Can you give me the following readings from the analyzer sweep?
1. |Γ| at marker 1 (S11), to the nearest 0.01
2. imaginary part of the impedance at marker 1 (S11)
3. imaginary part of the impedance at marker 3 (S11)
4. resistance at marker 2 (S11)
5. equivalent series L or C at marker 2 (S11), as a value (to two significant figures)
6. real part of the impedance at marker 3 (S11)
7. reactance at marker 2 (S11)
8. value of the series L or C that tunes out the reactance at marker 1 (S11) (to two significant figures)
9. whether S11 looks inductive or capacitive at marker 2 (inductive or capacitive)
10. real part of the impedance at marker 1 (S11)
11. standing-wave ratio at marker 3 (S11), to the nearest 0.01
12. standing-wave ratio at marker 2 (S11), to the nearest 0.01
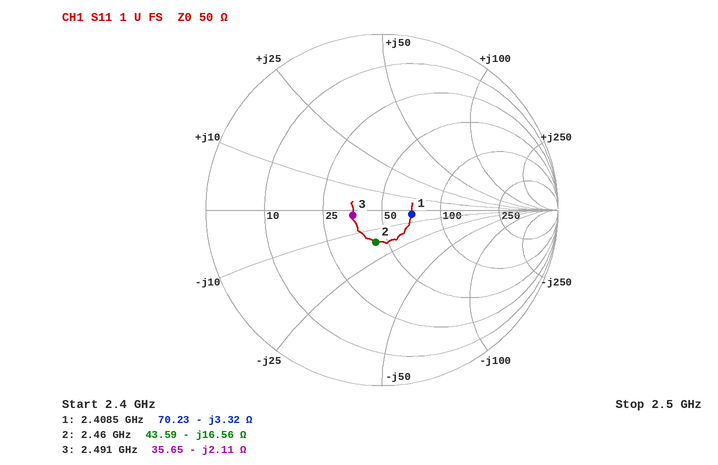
0.17
-3.32 Ω
-2.11 Ω
43.59 Ω
3.9 pF
35.65 Ω
-16.56 Ω
220 pH
capacitive
70.23 Ω
1.41
1.46
